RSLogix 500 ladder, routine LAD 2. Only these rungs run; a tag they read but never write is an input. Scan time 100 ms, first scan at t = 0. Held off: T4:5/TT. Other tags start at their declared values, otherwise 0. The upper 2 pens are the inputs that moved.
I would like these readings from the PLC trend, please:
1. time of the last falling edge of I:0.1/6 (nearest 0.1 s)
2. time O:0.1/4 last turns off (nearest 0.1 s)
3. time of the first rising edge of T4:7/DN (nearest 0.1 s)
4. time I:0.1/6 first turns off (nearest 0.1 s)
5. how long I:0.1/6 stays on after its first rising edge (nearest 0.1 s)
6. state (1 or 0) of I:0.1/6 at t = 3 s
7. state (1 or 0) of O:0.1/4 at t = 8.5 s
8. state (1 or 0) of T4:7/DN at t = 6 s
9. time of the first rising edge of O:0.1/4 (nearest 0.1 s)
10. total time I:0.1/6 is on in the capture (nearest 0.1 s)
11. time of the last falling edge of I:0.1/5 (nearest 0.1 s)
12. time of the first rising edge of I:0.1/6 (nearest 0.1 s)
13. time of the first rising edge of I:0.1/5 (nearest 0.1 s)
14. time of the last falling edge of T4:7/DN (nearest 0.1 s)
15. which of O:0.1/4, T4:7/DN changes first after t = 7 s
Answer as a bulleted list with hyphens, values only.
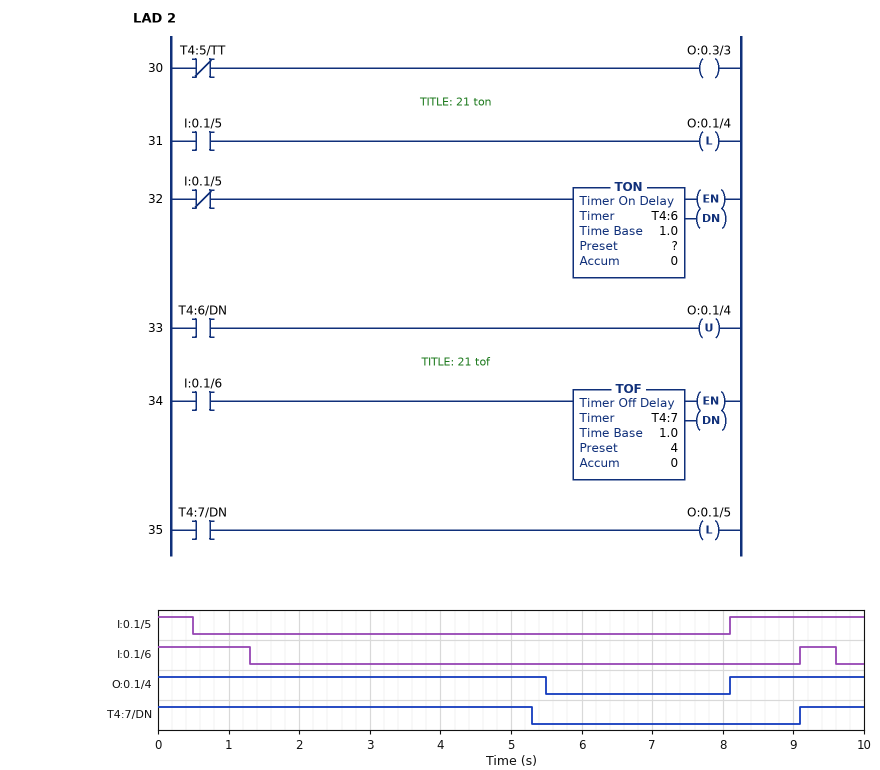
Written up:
- 9.6 s
- 5.5 s
- 9.1 s
- 1.3 s
- 0.5 s
- 0
- 1
- 0
- 8.1 s
- 1.8 s
- 0.5 s
- 9.1 s
- 8.1 s
- 5.3 s
- O:0.1/4
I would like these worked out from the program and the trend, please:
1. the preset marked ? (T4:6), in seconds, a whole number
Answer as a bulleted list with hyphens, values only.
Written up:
- 5 s
